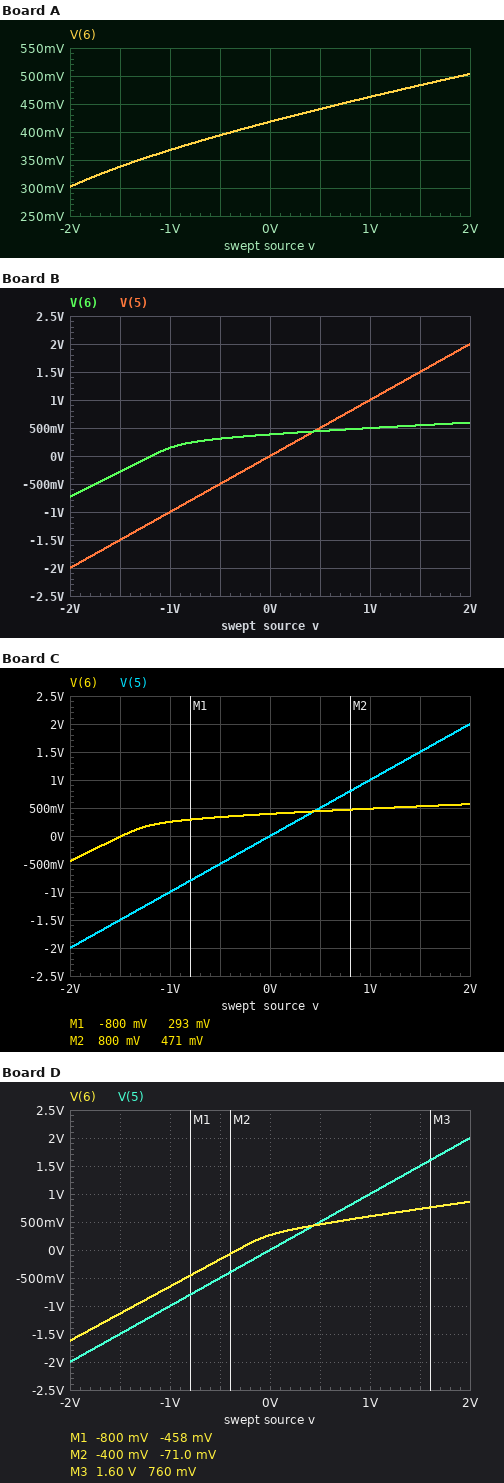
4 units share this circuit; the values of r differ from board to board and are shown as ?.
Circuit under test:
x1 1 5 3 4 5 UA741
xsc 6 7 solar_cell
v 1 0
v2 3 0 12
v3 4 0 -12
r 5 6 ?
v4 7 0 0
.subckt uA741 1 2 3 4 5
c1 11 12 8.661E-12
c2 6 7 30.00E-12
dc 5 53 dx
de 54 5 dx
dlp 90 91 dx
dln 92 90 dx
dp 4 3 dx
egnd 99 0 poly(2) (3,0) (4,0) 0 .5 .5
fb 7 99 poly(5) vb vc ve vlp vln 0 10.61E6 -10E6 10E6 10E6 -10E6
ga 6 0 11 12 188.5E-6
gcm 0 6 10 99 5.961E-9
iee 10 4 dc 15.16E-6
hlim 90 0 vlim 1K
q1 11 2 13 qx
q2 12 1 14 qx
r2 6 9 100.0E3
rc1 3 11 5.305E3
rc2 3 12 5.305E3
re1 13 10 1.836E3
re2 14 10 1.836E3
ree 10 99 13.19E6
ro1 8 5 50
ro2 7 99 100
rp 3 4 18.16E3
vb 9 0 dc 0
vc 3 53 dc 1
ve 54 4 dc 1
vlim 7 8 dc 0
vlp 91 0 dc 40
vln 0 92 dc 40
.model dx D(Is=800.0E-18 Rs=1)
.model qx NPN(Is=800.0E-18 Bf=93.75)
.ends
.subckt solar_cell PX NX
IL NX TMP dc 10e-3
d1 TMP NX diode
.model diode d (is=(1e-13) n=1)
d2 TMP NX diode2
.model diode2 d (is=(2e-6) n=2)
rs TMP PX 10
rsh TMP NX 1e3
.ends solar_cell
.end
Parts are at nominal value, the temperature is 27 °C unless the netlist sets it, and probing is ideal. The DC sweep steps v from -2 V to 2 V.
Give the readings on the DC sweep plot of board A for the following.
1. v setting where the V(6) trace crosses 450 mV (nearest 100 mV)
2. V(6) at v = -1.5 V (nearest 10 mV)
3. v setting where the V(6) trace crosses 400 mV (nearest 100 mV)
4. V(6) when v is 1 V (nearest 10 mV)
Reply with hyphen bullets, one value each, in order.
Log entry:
- 700 mV
- 340 mV
- -400 mV
- 460 mV
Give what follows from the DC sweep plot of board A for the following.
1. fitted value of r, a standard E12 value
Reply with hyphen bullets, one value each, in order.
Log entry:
- 330 Ω
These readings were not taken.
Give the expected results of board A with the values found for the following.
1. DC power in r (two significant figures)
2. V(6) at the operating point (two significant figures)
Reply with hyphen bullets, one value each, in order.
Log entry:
- 530 µW
- 420 mV
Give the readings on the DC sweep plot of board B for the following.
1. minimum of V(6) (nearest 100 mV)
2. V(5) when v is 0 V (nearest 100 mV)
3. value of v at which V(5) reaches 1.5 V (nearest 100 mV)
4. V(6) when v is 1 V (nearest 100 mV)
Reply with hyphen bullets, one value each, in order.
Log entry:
- -700 mV
- 0 V
- 1.5 V
- 500 mV
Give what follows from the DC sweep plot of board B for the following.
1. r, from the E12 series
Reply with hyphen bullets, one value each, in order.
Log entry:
- 120 Ω
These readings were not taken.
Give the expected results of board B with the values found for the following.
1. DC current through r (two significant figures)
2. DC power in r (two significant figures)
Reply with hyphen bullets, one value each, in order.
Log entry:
- 3.2 mA
- 1.2 mW
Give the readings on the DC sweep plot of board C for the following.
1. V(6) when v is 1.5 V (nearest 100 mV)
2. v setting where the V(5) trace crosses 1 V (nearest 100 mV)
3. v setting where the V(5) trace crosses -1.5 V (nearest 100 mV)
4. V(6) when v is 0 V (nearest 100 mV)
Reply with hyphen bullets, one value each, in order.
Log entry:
- 500 mV
- 1.0 V
- -1.5 V
- 400 mV
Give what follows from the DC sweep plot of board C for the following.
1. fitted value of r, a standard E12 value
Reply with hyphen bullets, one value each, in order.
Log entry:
- 150 Ω
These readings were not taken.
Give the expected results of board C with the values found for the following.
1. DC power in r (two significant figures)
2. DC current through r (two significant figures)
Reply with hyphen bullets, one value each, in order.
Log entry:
- 1.0 mW
- 2.6 mA
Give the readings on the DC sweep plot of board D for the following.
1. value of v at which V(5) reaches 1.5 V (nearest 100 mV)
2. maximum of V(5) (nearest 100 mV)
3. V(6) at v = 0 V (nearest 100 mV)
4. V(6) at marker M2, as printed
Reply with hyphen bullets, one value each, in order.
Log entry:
- 1.5 V
- 2.0 V
- 300 mV
- -71.0 mV
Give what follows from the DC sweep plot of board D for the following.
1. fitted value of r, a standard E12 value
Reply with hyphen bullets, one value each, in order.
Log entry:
- 33 Ω
